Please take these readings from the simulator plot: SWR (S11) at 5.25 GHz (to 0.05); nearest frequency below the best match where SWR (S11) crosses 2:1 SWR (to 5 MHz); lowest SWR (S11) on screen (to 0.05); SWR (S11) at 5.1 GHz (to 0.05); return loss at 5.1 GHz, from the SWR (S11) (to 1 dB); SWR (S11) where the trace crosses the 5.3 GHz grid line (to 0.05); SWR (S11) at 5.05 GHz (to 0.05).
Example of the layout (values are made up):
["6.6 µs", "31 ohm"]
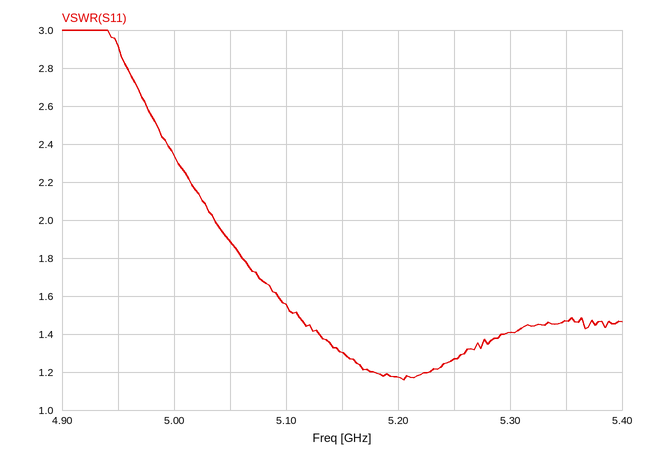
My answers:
["1.25", "5.035 GHz", "1.15", "1.55", "13 dB", "1.40", "1.90"]
